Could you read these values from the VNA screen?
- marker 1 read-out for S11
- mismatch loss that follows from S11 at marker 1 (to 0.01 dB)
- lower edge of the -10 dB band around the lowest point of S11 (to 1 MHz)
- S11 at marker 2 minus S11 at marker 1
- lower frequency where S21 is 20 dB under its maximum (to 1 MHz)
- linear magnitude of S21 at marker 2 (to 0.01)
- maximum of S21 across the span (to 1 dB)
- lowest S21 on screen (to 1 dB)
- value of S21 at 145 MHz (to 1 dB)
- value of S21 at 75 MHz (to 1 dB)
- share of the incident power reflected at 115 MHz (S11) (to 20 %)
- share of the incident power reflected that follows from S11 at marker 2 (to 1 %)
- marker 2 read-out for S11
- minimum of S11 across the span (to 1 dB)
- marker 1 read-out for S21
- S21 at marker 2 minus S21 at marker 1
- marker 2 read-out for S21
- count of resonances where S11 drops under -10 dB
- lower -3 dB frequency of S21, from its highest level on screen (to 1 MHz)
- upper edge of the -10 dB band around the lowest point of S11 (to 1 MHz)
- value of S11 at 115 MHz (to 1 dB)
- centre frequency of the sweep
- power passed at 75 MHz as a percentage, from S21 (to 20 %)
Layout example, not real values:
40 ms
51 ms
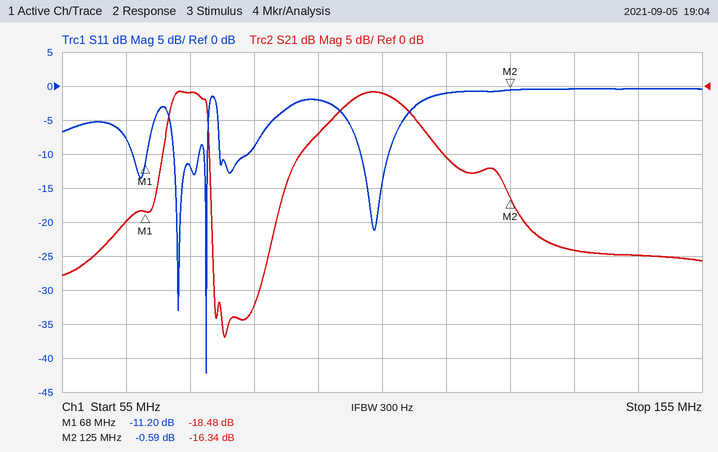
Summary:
-11.20 dB
0.34 dB
77 MHz
10.61 dB
64 MHz
0.15
-1 dB
-37 dB
-25 dB
-1 dB
80 %
87 %
-0.59 dB
-42 dB
-18.48 dB
2.14 dB
-16.34 dB
5
72 MHz
78 MHz
-1 dB
105 MHz
80 %
